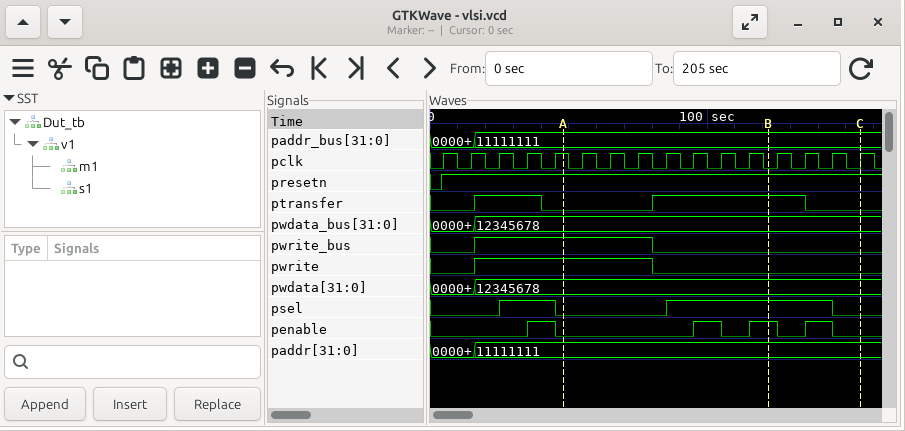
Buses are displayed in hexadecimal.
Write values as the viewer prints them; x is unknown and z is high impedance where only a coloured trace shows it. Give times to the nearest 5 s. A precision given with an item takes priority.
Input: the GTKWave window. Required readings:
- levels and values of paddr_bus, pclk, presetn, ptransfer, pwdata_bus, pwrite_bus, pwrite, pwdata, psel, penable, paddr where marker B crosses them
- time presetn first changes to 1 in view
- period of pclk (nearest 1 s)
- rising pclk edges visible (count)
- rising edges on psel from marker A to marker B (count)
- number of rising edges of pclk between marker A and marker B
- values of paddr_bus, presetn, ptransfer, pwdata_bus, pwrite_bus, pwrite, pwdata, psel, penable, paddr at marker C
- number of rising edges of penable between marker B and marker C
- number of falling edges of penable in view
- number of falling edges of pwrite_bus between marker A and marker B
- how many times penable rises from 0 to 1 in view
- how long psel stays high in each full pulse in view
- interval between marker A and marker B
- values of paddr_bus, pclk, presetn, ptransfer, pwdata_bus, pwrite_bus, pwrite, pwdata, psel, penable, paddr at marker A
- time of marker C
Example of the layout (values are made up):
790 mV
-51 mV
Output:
paddr_bus=11111111, pclk=0, presetn=1, ptransfer=1, pwdata_bus=12345678, pwrite_bus=0, pwrite=0, pwdata=12345678, psel=1, penable=1, paddr=11111111
5 s
10 s
16
1
7
paddr_bus=11111111, presetn=1, ptransfer=0, pwdata_bus=12345678, pwrite_bus=0, pwrite=0, pwdata=12345678, psel=0, penable=0, paddr=11111111
1
4
1
4
20 s, 60 s
75 s
paddr_bus=11111111, pclk=1, presetn=1, ptransfer=0, pwdata_bus=12345678, pwrite_bus=1, pwrite=1, pwdata=12345678, psel=0, penable=0, paddr=11111111
155 s
